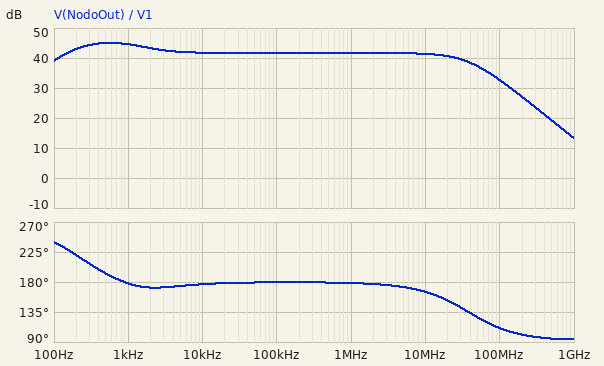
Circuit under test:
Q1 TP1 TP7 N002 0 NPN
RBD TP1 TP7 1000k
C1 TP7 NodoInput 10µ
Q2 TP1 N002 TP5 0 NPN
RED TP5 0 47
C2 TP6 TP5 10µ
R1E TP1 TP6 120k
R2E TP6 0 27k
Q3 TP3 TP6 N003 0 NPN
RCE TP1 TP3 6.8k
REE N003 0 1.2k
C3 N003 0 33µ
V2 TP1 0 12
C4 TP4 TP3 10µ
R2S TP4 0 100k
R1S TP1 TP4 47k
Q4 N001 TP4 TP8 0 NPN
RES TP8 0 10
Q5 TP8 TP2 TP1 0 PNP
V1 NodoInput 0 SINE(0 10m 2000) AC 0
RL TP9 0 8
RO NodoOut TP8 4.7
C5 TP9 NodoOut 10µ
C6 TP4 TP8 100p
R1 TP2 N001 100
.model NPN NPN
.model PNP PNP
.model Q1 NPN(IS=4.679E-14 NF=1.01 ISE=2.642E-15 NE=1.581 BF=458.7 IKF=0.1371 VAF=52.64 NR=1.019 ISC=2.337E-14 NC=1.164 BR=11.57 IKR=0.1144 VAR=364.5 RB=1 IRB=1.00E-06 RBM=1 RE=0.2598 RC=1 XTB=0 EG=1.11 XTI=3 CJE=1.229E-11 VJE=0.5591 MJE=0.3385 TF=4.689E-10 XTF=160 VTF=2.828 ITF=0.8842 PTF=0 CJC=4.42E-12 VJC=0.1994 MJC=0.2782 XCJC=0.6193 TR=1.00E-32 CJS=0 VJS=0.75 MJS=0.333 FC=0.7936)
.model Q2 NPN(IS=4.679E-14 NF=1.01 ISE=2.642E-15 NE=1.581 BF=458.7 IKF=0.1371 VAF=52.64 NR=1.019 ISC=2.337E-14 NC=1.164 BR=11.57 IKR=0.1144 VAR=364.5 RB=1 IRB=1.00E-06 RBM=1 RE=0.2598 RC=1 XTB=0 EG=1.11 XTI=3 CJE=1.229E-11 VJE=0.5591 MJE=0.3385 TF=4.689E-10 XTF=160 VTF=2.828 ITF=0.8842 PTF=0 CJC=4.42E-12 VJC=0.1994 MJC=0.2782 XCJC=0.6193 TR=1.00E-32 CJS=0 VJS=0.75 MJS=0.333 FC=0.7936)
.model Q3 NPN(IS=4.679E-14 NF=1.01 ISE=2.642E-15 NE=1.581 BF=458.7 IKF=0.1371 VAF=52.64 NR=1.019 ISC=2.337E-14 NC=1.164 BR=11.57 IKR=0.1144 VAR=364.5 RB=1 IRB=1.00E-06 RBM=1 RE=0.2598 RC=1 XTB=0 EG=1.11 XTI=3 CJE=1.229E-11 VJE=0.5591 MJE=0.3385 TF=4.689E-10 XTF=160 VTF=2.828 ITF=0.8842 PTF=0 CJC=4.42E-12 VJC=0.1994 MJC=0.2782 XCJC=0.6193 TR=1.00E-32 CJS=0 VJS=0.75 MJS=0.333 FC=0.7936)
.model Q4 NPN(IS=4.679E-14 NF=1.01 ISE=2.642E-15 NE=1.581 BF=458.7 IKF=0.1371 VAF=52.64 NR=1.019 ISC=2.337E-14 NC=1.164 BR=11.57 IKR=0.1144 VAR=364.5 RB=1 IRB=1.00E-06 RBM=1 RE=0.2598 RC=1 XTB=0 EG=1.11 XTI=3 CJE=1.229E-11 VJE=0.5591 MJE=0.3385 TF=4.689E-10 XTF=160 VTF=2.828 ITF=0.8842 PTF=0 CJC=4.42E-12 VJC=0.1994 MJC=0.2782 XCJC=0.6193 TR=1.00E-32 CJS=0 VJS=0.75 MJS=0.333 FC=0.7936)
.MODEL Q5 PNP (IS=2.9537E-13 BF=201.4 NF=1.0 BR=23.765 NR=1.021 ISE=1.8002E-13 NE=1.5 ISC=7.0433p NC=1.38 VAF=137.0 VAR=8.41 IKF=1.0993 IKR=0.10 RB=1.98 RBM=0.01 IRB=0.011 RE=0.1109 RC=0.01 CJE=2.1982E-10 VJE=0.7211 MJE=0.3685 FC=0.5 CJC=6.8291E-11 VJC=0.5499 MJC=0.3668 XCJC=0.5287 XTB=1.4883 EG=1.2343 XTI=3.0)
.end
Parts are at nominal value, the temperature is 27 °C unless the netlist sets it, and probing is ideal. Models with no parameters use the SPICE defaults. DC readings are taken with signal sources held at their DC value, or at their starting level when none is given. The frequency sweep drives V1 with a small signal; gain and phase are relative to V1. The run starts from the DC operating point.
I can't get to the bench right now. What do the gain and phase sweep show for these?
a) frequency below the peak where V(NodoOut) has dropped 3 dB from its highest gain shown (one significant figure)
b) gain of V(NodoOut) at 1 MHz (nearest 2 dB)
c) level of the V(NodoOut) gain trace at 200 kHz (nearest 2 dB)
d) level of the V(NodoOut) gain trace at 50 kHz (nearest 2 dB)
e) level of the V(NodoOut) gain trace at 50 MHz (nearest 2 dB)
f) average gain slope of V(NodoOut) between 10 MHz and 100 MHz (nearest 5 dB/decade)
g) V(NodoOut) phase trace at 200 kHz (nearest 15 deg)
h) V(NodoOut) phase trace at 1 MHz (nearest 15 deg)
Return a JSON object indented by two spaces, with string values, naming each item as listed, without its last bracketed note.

{
  "frequency below the peak where V(NodoOut) has dropped 3 dB from its highest gain shown": "200 Hz",
  "gain of V(NodoOut) at 1 MHz": "42 dB",
  "level of the V(NodoOut) gain trace at 200 kHz": "42 dB",
  "level of the V(NodoOut) gain trace at 50 kHz": "42 dB",
  "level of the V(NodoOut) gain trace at 50 MHz": "38 dB",
  "average gain slope of V(NodoOut) between 10 MHz and 100 MHz": "-10 dB/decade",
  "V(NodoOut) phase trace at 200 kHz": "180 deg",
  "V(NodoOut) phase trace at 1 MHz": "180 deg"
}
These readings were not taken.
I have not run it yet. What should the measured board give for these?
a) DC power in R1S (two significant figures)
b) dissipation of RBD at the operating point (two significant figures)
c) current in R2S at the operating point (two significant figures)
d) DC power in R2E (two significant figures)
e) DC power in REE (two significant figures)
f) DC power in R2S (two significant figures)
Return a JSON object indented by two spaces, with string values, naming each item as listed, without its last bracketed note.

{
  "DC power in R1S": "670 µW",
  "dissipation of RBD at the operating point": "49 µW",
  "current in R2S at the operating point": "64 µA",
  "DC power in R2E": "150 µW",
  "DC power in REE": "1.2 mW",
  "DC power in R2S": "410 µW"
}
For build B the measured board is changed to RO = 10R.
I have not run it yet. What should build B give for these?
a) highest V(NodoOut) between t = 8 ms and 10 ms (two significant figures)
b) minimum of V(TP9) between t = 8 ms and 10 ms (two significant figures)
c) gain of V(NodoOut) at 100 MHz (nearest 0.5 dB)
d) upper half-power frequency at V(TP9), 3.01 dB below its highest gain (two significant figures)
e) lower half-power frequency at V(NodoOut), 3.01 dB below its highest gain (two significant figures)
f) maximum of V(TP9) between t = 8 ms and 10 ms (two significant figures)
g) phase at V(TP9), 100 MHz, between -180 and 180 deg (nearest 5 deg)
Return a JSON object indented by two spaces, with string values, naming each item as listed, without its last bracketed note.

{
  "highest V(NodoOut) between t = 8 ms and 10 ms": "6.6 V",
  "minimum of V(TP9) between t = 8 ms and 10 ms": "-850 mV",
  "gain of V(NodoOut) at 100 MHz": "30.5 dB",
  "upper half-power frequency at V(TP9), 3.01 dB below its highest gain": "43 MHz",
  "lower half-power frequency at V(NodoOut), 3.01 dB below its highest gain": "150 Hz",
  "maximum of V(TP9) between t = 8 ms and 10 ms": "720 mV",
  "phase at V(TP9), 100 MHz, between -180 and 180 deg": "115 deg"
}
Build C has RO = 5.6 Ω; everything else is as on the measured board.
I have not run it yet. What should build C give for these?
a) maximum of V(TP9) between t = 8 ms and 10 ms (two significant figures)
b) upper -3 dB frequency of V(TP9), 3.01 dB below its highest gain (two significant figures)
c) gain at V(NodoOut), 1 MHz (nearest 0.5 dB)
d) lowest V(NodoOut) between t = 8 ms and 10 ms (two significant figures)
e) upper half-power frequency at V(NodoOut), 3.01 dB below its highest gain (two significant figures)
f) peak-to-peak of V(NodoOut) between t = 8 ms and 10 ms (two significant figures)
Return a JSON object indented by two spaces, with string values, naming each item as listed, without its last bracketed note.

{
  "maximum of V(TP9) between t = 8 ms and 10 ms": "900 mV",
  "upper -3 dB frequency of V(TP9), 3.01 dB below its highest gain": "39 MHz",
  "gain at V(NodoOut), 1 MHz": "41.0 dB",
  "lowest V(NodoOut) between t = 8 ms and 10 ms": "4.1 V",
  "upper half-power frequency at V(NodoOut), 3.01 dB below its highest gain": "3.4 kHz",
  "peak-to-peak of V(NodoOut) between t = 8 ms and 10 ms": "2.7 V"
}
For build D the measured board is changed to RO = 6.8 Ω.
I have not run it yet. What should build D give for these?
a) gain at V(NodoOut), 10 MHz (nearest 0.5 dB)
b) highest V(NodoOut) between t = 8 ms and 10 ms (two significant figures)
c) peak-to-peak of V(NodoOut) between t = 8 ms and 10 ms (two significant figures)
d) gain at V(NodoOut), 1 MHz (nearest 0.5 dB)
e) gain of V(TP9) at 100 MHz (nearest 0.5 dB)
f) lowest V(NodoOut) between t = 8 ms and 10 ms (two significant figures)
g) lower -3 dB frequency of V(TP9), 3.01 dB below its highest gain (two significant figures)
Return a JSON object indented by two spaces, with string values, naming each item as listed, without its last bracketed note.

{
  "gain at V(NodoOut), 10 MHz": "40.0 dB",
  "highest V(NodoOut) between t = 8 ms and 10 ms": "6.8 V",
  "peak-to-peak of V(NodoOut) between t = 8 ms and 10 ms": "2.6 V",
  "gain at V(NodoOut), 1 MHz": "40.5 dB",
  "gain of V(TP9) at 100 MHz": "32.0 dB",
  "lowest V(NodoOut) between t = 8 ms and 10 ms": "4.2 V",
  "lower -3 dB frequency of V(TP9), 3.01 dB below its highest gain": "1.1 kHz"
}
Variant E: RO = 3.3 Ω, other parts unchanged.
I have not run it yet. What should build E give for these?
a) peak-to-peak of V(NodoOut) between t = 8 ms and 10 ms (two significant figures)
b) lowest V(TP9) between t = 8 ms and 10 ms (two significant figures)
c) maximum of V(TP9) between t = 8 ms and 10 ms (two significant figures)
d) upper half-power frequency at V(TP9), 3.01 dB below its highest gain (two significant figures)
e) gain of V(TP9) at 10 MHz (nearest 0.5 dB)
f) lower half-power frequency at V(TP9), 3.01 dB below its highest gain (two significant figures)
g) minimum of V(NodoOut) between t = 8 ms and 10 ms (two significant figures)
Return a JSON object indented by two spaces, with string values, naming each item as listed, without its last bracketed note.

{
  "peak-to-peak of V(NodoOut) between t = 8 ms and 10 ms": "3.1 V",
  "lowest V(TP9) between t = 8 ms and 10 ms": "-1.2 V",
  "maximum of V(TP9) between t = 8 ms and 10 ms": "1.0 V",
  "upper half-power frequency at V(TP9), 3.01 dB below its highest gain": "36 MHz",
  "gain of V(TP9) at 10 MHz": "42.5 dB",
  "lower half-power frequency at V(TP9), 3.01 dB below its highest gain": "1.4 kHz",
  "minimum of V(NodoOut) between t = 8 ms and 10 ms": "3.9 V"
}
